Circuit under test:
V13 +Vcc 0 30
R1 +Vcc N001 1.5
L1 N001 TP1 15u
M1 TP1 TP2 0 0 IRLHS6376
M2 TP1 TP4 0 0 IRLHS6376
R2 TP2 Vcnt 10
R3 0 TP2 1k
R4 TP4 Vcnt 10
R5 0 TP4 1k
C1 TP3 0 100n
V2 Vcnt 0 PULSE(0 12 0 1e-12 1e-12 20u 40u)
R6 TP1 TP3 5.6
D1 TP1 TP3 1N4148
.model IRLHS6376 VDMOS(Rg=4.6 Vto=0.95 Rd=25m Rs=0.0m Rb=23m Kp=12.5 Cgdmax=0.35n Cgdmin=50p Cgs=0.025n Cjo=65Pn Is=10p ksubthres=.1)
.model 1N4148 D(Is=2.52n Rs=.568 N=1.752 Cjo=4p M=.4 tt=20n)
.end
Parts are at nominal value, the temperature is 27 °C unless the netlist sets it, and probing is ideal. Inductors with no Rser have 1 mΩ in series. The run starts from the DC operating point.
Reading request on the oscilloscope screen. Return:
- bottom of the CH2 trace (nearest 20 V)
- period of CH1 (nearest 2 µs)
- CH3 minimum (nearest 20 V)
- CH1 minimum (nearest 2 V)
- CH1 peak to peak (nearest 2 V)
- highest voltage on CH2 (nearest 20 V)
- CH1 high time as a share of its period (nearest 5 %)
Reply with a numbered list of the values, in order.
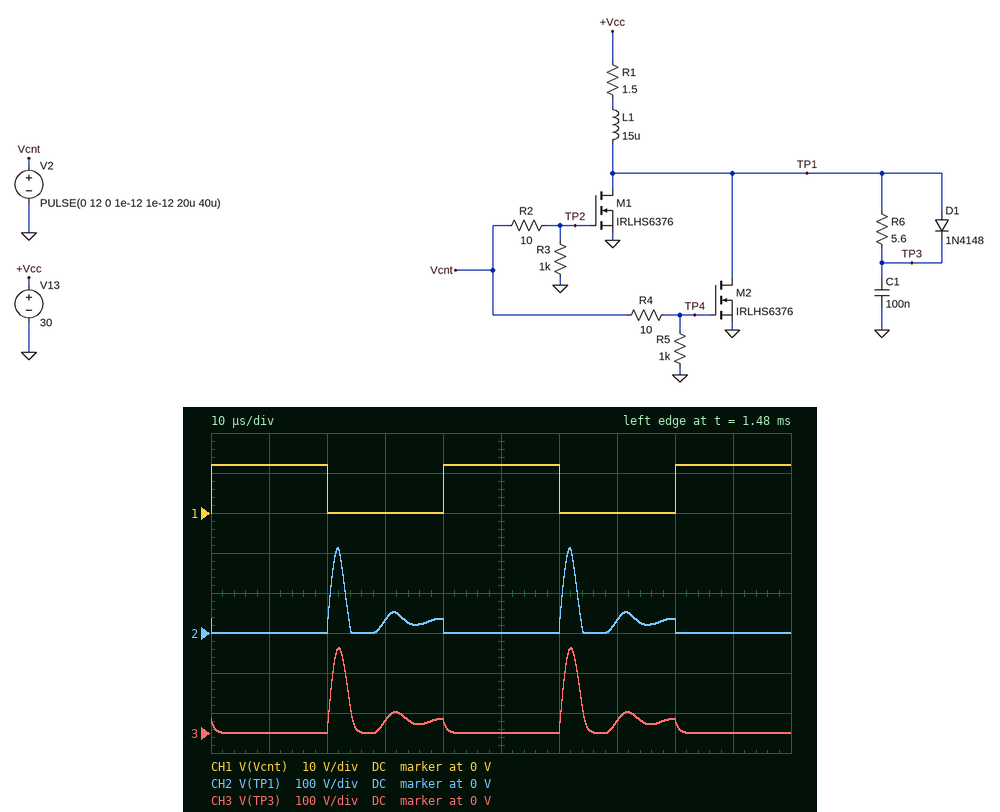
1. 0 V
2. 40 µs
3. 0 V
4. 0 V
5. 12 V
6. 220 V
7. 50 %
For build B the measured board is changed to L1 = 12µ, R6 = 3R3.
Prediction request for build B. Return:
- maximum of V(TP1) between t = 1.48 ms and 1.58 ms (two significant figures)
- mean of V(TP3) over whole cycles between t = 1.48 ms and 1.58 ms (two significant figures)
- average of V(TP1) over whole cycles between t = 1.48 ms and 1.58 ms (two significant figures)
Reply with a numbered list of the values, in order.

1. 200 V
2. 23 V
3. 21 V
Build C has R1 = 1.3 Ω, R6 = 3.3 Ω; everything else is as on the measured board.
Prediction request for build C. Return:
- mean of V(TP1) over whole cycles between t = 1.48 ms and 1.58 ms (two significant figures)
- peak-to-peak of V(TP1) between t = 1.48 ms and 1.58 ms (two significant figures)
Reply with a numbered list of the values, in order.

1. 23 V
2. 240 V
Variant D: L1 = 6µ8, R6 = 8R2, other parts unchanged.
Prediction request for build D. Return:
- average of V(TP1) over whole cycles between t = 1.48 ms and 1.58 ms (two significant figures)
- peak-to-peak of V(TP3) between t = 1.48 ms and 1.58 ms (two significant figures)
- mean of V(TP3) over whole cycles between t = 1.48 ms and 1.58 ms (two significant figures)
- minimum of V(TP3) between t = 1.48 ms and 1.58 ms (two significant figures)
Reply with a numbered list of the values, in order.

1. 18 V
2. 160 V
3. 22 V
4. 240 mV
